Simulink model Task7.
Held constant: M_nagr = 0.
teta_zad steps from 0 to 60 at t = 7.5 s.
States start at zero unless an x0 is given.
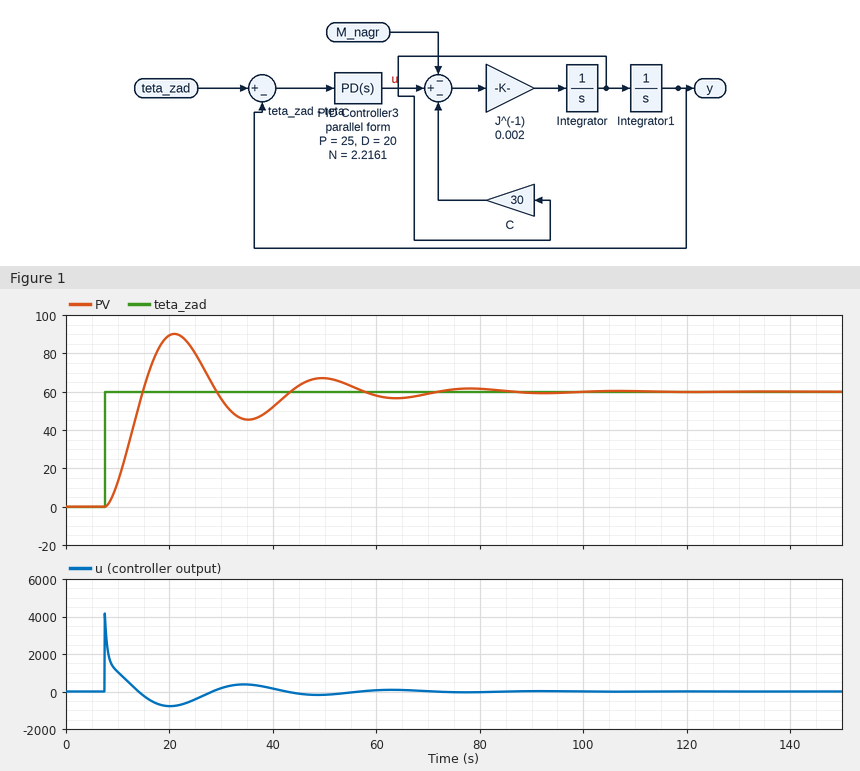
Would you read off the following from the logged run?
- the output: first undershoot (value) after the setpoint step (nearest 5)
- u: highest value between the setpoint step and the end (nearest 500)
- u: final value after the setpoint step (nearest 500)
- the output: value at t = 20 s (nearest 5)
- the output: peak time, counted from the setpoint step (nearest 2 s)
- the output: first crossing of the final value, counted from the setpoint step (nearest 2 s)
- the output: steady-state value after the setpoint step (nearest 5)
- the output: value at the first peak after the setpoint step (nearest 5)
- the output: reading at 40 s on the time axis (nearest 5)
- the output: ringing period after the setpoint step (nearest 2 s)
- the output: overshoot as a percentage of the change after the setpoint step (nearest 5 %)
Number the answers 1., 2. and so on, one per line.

1. 45
2. 4000
3. 0
4. 90
5. 14 s
6. 8 s
7. 60
8. 90
9. 50
10. 28 s
11. 50 %
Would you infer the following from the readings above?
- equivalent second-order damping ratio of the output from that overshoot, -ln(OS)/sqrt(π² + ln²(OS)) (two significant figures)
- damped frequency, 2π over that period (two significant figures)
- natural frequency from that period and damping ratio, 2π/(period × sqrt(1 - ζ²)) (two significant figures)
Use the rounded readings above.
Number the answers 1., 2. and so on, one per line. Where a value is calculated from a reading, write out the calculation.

1. ln(0.5) = -0.693; 0.693 / sqrt(9.870 + 0.480) = 0.22
2. 2π / 28 = 0.22 rad/s
3. 2π / (28 × sqrt(1 - 0.22²)) = 0.23 rad/s
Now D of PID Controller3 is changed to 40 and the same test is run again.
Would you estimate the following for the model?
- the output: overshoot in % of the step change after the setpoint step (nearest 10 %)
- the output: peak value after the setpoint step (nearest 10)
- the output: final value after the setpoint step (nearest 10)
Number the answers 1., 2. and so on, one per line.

1. 40 %
2. 80
3. 60
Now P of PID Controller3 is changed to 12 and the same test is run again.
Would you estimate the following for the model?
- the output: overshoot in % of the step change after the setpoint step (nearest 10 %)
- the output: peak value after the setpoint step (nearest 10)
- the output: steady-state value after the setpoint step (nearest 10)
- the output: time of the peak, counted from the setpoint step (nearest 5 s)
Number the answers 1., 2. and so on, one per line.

1. 40 %
2. 80
3. 60
4. 20 s
